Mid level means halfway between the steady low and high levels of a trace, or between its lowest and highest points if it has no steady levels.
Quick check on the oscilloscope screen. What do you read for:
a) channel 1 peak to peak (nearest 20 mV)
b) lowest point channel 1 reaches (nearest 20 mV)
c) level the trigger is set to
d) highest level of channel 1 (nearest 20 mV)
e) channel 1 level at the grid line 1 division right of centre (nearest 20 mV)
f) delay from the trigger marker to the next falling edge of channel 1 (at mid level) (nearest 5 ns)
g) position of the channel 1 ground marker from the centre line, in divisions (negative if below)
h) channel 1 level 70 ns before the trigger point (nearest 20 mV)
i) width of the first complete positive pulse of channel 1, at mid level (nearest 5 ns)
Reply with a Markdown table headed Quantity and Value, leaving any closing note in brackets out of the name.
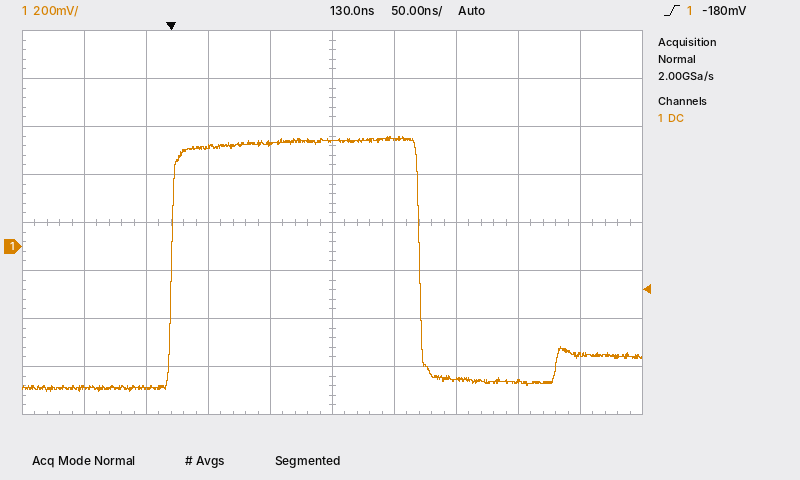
| Quantity | Value |
|---|---|
| channel 1 peak to peak | 1.06 V |
| lowest point channel 1 reaches | -600 mV |
| level the trigger is set to | -180 mV |
| highest level of channel 1 | 460 mV |
| channel 1 level at the grid line 1 division right of centre | 440 mV |
| delay from the trigger marker to the next falling edge of channel 1 (at mid level) | 200 ns |
| position of the channel 1 ground marker from the centre line, in divisions | -0.5 div |
| channel 1 level 70 ns before the trigger point | -580 mV |
| width of the first complete positive pulse of channel 1, at mid level | 200 ns |
